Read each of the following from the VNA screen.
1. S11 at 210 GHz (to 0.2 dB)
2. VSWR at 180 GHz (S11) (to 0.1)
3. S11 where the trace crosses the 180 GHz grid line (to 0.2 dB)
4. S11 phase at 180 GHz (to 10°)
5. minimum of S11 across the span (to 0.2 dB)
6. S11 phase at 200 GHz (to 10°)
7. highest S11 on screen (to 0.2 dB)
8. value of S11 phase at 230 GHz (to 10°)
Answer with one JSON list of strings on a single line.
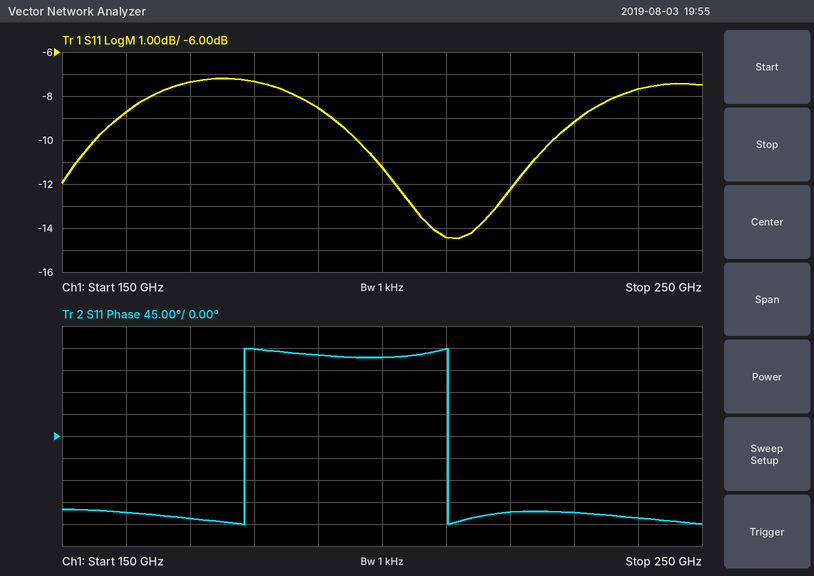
["-14.4 dB", "2.5", "-7.4 dB", "180°", "-14.4 dB", "160°", "-7.2 dB", "-160°"]
